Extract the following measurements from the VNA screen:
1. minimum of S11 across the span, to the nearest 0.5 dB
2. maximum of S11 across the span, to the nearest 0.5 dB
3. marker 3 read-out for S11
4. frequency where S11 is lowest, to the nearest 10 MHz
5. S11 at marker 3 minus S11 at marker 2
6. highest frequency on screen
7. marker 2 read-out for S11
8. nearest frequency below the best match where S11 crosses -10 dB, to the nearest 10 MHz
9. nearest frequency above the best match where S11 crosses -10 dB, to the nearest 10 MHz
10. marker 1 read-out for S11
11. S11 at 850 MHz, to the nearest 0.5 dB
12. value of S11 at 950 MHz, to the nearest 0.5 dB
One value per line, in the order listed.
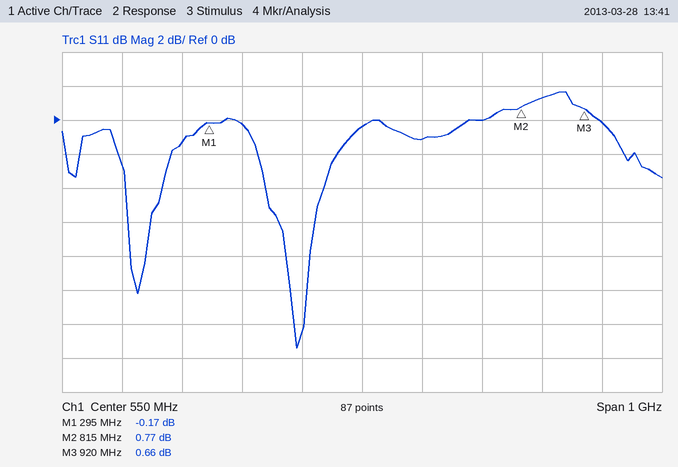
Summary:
-13.5 dB
1.5 dB
0.66 dB
440 MHz
-0.11 dB
1.05 GHz
0.77 dB
430 MHz
460 MHz
-0.17 dB
1.5 dB
0.0 dB
